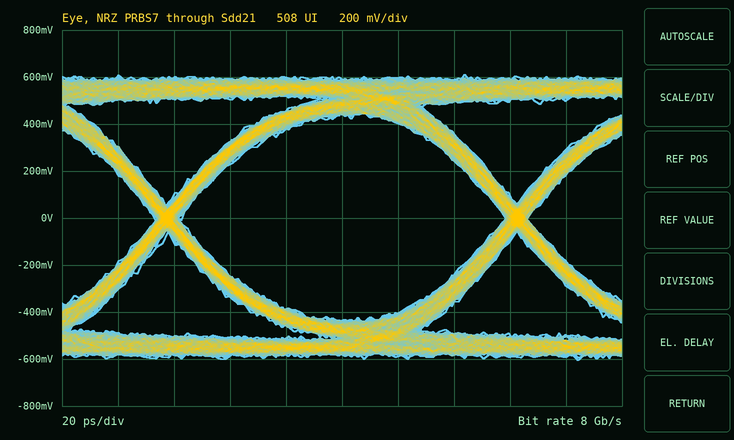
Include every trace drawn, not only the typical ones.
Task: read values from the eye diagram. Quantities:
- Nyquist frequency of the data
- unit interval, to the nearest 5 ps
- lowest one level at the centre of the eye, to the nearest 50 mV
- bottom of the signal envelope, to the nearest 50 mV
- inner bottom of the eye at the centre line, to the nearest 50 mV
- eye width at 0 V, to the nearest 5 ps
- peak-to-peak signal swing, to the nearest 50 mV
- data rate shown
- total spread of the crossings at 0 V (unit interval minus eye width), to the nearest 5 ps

4 GHz
125 ps
450 mV
-600 mV
-450 mV
115 ps
1.20 V
8 Gb/s
10 ps
